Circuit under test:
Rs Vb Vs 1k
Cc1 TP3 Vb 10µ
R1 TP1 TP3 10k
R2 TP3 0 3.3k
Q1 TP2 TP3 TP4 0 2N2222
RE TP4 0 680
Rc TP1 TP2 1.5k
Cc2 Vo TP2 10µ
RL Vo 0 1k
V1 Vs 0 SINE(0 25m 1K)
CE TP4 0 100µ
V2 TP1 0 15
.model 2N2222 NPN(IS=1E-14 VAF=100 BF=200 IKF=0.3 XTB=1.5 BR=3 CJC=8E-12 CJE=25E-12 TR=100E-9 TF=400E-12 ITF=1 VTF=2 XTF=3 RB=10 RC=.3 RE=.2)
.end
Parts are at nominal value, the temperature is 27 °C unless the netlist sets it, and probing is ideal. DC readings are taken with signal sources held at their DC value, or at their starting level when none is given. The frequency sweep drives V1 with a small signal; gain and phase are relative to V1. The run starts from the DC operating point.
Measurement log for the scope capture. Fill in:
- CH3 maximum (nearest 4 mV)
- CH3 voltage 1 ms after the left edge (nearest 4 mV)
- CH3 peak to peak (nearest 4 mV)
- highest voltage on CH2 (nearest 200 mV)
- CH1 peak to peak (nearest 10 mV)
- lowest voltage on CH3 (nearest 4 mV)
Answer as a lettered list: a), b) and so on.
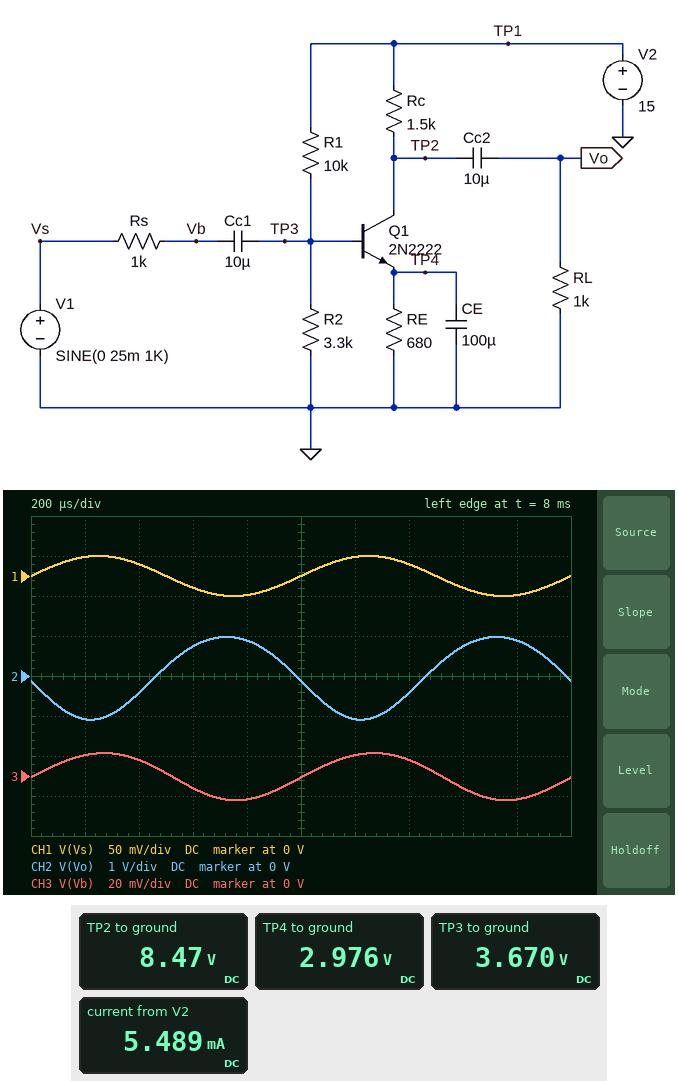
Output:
a) 12 mV
b) 0 V
c) 24 mV
d) 1.0 V
e) 50 mV
f) -12 mV
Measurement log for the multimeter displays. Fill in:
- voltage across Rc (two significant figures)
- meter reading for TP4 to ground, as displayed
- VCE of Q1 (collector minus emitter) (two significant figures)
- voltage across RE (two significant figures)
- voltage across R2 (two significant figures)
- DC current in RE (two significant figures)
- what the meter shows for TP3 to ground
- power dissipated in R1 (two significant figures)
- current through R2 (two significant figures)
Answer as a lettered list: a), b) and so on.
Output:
a) 6.5 V
b) 2.976 V
c) 5.5 V
d) 3.0 V
e) 3.7 V
f) 4.4 mA
g) 3.670 V
h) 13 mW
i) 1.1 mA
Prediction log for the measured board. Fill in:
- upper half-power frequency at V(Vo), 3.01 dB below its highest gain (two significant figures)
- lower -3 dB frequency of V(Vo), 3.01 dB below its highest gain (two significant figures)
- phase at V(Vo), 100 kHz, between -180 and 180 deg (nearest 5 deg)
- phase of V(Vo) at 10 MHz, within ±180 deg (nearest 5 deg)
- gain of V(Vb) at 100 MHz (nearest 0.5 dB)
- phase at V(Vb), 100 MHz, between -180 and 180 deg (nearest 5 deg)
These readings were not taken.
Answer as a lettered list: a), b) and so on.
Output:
a) 690 kHz
b) 170 Hz
c) 170 deg
d) 90 deg
e) -37.0 dB
f) -15 deg
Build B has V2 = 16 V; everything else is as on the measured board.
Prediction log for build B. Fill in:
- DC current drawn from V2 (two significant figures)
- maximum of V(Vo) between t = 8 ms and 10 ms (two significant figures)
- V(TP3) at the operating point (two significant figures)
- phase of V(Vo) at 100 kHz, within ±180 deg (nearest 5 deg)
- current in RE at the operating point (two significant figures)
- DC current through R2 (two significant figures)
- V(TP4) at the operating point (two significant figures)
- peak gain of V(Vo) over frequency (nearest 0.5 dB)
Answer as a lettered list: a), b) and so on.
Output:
a) 5.9 mA
b) 1.0 V
c) 3.9 V
d) 170 deg
e) 4.7 mA
f) 1.2 mA
g) 3.2 V
h) 33.0 dB
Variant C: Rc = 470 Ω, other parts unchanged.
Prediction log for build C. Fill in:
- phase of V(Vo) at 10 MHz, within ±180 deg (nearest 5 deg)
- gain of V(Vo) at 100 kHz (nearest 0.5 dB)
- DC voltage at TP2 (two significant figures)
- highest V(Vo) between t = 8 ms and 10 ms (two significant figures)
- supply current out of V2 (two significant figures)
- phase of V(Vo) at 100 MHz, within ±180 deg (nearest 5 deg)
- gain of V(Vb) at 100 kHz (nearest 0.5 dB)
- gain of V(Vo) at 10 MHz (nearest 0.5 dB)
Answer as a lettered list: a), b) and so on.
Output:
a) 95 deg
b) 27.5 dB
c) 13 V
d) 530 mV
e) 5.5 mA
f) 75 deg
g) -6.5 dB
h) 9.0 dB
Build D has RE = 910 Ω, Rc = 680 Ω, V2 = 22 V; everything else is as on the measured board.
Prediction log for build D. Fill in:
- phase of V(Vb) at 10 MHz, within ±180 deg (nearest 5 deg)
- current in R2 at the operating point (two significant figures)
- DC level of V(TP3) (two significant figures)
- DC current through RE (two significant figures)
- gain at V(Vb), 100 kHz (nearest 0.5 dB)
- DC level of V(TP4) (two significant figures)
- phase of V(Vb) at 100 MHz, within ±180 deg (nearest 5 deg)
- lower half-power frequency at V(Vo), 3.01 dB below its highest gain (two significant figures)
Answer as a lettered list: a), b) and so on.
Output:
a) -70 deg
b) 1.6 mA
c) 5.4 V
d) 5.2 mA
e) -7.0 dB
f) 4.7 V
g) -20 deg
h) 190 Hz
